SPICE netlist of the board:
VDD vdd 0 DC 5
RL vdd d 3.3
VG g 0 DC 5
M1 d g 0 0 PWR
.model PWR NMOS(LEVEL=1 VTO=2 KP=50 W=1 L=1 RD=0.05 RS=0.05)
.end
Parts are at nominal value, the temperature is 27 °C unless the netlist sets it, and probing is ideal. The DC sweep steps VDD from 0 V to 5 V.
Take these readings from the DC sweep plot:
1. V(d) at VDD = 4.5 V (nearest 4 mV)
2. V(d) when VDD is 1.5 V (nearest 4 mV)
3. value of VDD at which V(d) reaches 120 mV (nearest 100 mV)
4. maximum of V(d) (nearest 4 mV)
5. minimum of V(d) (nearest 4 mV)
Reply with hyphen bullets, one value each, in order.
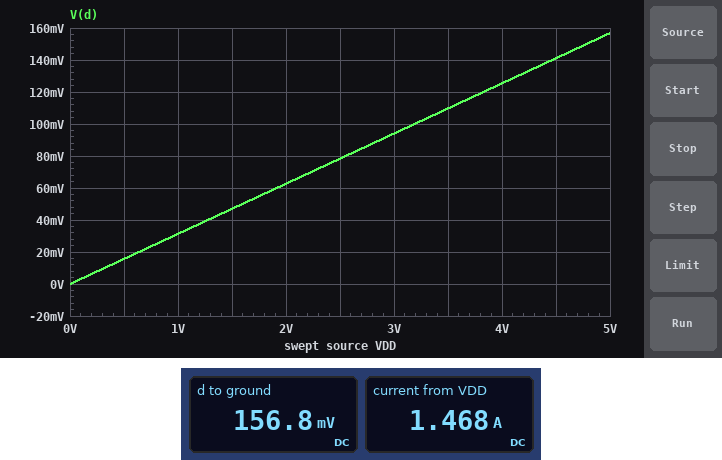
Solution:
- 140 mV
- 48 mV
- 3.8 V
- 156 mV
- 0 V
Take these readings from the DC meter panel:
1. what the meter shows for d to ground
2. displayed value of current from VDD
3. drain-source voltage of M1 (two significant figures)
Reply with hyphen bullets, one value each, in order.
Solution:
- 156.8 mV
- 1.468 A
- 160 mV
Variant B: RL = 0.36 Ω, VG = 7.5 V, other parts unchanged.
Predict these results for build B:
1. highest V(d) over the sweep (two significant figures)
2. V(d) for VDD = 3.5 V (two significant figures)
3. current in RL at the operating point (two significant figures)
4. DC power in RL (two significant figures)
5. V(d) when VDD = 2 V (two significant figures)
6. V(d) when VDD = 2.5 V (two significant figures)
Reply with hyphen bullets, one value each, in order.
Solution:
- 1.1 V
- 780 mV
- 11 A
- 42 W
- 450 mV
- 560 mV
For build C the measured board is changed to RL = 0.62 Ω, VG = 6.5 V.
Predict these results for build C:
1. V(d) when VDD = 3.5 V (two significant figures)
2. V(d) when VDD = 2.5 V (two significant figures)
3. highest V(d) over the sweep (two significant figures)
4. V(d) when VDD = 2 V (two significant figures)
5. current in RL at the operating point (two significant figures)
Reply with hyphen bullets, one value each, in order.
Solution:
- 510 mV
- 360 mV
- 720 mV
- 290 mV
- 6.9 A
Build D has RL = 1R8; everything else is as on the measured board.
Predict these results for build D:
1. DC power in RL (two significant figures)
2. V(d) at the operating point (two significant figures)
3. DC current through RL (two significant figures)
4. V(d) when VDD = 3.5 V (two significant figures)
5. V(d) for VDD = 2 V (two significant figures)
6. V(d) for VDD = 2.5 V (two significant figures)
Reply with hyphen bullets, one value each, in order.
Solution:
- 12 W
- 280 mV
- 2.6 A
- 200 mV
- 110 mV
- 140 mV
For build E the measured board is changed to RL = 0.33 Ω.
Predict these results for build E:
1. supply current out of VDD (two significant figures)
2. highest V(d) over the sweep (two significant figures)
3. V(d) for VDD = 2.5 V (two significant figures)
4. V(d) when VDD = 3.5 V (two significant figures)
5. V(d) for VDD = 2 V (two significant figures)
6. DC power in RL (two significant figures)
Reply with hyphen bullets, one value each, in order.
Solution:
- 11 A
- 1.2 V
- 610 mV
- 860 mV
- 490 mV
- 43 W
